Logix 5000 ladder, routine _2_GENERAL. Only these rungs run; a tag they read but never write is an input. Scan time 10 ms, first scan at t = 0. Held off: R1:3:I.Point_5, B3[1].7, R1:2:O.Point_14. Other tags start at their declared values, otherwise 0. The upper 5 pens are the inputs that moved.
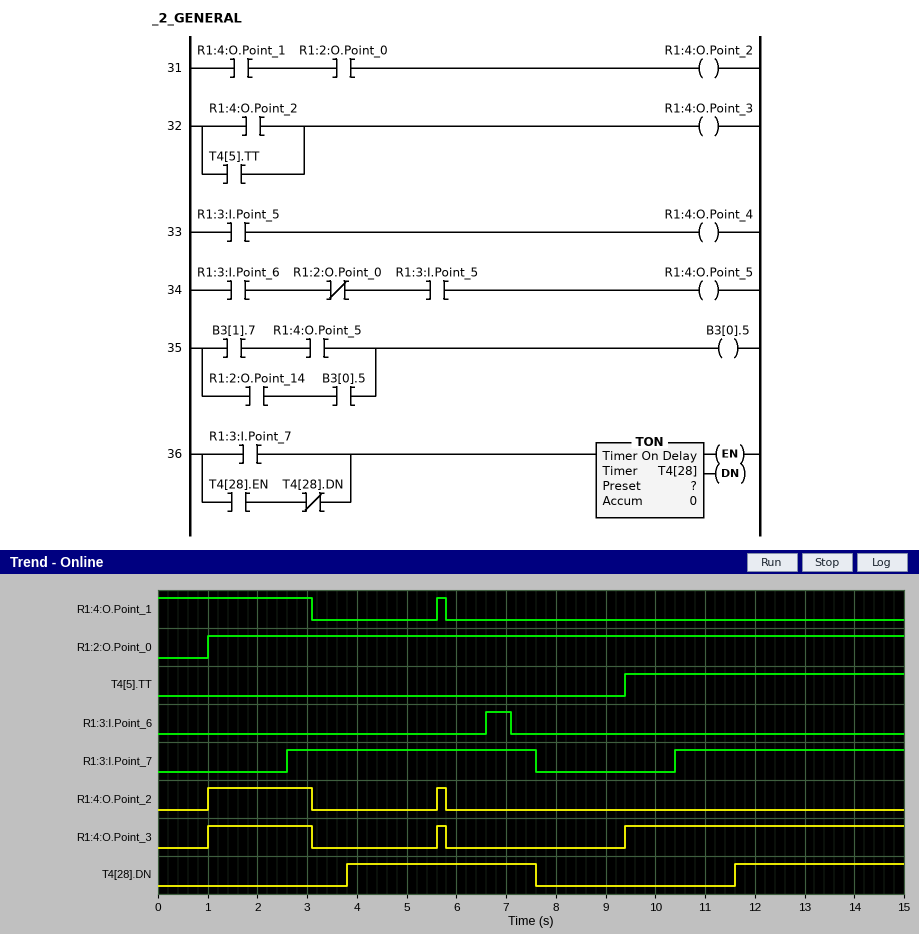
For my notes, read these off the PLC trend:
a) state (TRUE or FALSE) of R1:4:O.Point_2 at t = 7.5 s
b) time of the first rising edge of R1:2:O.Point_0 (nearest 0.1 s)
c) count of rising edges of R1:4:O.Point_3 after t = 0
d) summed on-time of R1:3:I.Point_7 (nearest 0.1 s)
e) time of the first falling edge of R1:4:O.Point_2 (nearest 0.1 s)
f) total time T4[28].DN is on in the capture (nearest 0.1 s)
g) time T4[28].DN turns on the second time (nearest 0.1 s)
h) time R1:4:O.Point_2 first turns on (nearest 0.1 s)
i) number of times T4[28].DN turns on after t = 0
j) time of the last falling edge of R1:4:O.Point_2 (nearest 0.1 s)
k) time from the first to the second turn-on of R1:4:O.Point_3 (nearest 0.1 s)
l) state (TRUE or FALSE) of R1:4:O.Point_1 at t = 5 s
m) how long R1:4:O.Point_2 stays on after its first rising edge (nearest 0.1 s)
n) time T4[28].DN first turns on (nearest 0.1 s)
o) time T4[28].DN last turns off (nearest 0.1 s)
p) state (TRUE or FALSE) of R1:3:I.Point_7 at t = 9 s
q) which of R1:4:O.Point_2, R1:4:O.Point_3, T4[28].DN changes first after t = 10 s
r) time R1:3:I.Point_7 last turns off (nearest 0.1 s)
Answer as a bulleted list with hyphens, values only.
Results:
- FALSE
- 1.0 s
- 3
- 9.6 s
- 3.1 s
- 7.2 s
- 11.6 s
- 1.0 s
- 2
- 5.8 s
- 4.6 s
- FALSE
- 2.1 s
- 3.8 s
- 7.6 s
- FALSE
- T4[28].DN
- 7.6 s
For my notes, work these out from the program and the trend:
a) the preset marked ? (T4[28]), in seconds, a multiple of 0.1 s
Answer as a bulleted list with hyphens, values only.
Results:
- 1.2 s
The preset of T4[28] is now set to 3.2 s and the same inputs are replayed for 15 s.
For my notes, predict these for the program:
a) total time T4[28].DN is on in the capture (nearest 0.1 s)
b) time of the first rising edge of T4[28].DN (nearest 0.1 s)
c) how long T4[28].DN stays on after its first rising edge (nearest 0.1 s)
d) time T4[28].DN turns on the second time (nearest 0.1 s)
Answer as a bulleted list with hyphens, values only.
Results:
- 3.2 s
- 5.8 s
- 1.8 s
- 13.6 s
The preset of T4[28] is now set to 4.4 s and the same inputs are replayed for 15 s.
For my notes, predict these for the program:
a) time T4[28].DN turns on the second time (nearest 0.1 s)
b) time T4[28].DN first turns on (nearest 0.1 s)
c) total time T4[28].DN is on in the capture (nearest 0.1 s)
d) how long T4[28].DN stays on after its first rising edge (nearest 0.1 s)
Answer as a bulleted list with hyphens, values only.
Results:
- 14.8 s
- 7.0 s
- 0.8 s
- 0.6 s
